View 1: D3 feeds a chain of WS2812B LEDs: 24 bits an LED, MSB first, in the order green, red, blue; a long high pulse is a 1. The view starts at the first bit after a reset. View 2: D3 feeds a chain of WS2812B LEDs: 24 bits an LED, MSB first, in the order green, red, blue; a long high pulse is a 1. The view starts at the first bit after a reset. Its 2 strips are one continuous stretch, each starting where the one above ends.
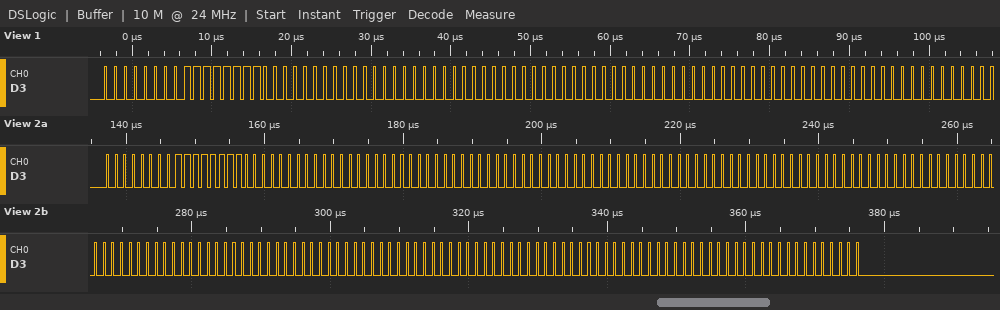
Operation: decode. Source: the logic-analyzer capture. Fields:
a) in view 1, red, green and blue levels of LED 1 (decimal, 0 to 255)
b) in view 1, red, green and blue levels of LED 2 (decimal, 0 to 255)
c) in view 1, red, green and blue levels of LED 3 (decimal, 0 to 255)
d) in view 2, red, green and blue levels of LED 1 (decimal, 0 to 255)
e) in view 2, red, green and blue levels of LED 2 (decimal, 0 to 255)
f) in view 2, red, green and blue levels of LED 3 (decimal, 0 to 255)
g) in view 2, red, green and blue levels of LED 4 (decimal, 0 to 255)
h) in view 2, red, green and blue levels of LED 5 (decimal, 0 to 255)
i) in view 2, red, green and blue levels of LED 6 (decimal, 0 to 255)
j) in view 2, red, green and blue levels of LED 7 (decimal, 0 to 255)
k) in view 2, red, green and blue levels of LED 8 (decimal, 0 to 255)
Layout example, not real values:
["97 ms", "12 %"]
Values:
["255, 0, 0", "0, 0, 0", "0, 0, 0", "255, 0, 0", "0, 0, 0", "0, 0, 0", "0, 0, 0", "0, 0, 0", "0, 0, 0", "0, 0, 0", "0, 0, 0"]
